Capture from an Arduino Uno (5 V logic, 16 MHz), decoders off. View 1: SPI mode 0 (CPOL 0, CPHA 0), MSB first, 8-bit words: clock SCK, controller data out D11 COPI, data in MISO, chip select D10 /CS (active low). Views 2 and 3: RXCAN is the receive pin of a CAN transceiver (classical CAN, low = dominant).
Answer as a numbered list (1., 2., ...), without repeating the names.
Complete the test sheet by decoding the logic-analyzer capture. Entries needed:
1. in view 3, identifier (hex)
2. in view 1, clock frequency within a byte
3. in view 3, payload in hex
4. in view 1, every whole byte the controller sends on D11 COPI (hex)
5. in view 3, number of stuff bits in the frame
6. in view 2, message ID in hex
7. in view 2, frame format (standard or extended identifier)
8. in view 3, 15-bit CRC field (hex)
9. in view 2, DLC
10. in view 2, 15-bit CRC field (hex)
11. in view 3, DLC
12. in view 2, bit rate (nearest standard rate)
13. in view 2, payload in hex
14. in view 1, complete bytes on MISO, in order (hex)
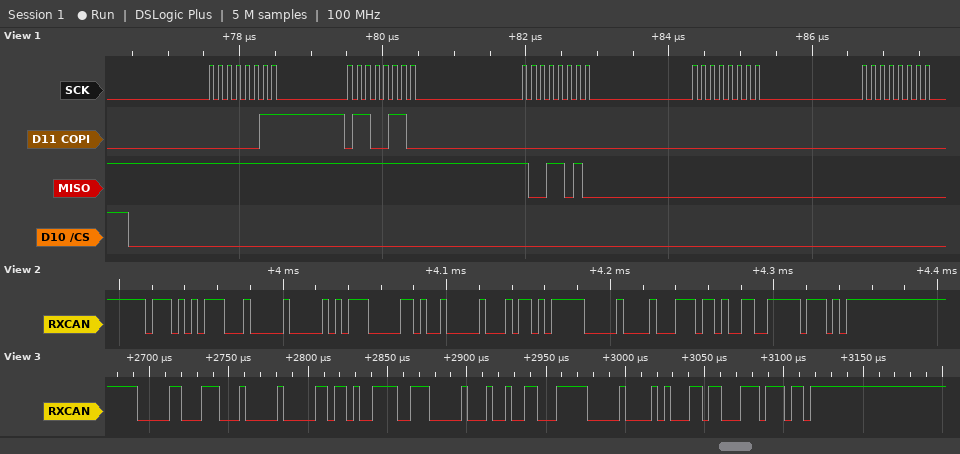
1. 0x047
2. 8 MHz
3. 01 69 E7 00 93 1F 00 A3
4. 03 66 00 00 00
5. 6
6. 0x757
7. standard
8. 0x31DD
9. 8
10. 0x19FE
11. 8
12. 250 kbit/s
13. 00 B8 29 00 B5 F0 08 ED
14. FF FF 9A 00 00
